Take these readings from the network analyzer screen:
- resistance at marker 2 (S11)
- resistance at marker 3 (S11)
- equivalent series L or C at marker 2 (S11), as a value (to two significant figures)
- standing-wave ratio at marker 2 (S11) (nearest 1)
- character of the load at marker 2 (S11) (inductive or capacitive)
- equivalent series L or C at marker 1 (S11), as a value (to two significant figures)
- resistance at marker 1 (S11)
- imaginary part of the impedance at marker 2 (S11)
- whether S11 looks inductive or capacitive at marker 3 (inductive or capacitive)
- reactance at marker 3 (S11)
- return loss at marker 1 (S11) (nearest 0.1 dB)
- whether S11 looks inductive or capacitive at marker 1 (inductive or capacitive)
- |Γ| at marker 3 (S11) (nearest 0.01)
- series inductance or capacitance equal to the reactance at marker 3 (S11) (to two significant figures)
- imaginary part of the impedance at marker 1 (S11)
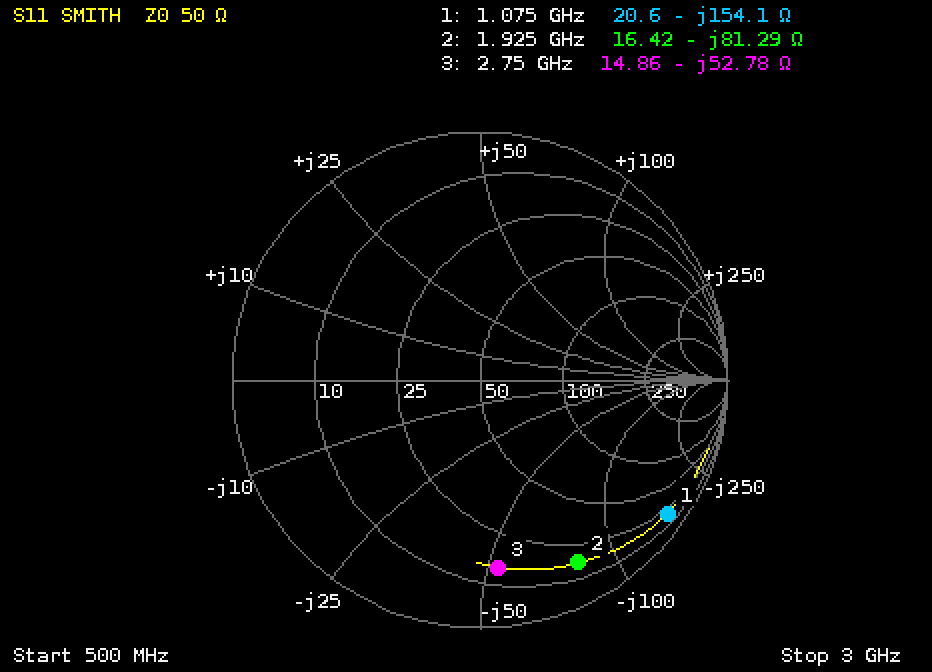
16.42 Ω
14.86 Ω
1.0 pF
11
capacitive
960 fF
20.6 Ω
-81.29 Ω
capacitive
-52.78 Ω
0.7 dB
capacitive
0.76
1.1 pF
-154.1 Ω
